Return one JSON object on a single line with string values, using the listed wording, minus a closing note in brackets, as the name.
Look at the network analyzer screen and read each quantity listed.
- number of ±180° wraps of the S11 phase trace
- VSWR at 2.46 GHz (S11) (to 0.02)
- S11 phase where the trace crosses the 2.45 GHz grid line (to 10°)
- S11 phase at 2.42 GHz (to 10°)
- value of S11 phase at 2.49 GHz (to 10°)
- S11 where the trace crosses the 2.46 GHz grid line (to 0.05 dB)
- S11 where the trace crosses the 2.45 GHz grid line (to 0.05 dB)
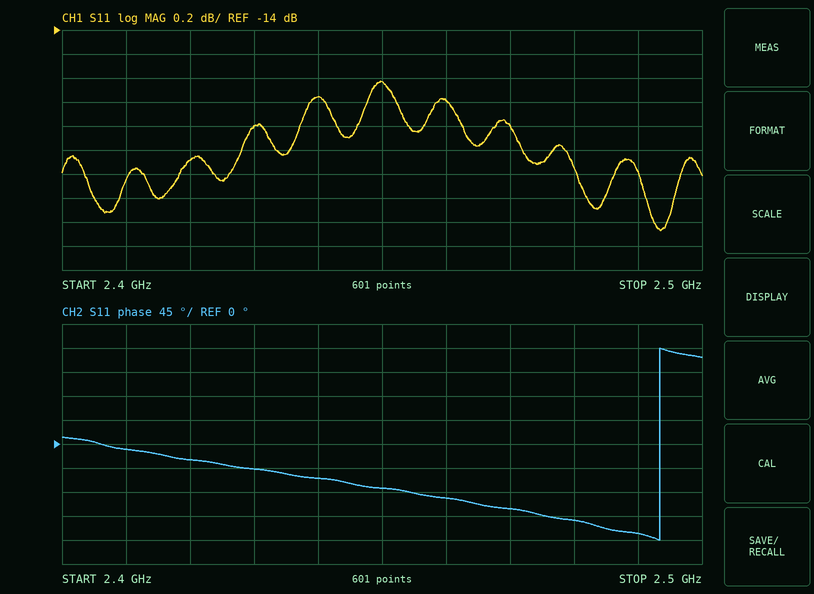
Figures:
{"number of ±180° wraps of the S11 phase trace": "1", "VSWR at 2.46 GHz (S11)": "1.46", "S11 phase where the trace crosses the 2.45 GHz grid line": "-80°", "S11 phase at 2.42 GHz": "-30°", "value of S11 phase at 2.49 GHz": "-170°", "S11 where the trace crosses the 2.46 GHz grid line": "-14.60 dB", "S11 where the trace crosses the 2.45 GHz grid line": "-14.45 dB"}
